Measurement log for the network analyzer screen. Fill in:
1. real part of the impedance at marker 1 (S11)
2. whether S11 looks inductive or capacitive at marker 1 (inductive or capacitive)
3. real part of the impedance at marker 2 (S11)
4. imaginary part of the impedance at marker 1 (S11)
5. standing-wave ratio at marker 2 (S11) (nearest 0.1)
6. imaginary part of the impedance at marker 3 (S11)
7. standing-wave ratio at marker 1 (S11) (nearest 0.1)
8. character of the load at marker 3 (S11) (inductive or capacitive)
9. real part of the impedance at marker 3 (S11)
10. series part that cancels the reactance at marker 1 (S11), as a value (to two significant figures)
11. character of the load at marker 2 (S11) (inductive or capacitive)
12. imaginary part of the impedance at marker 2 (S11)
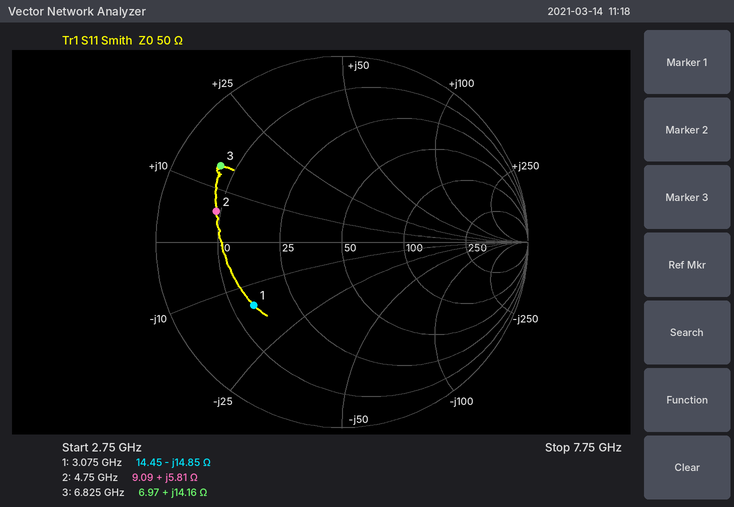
14.45 Ω
capacitive
9.09 Ω
-14.85 Ω
5.6
+14.16 Ω
3.8
inductive
6.97 Ω
770 pH
inductive
+5.81 Ω
